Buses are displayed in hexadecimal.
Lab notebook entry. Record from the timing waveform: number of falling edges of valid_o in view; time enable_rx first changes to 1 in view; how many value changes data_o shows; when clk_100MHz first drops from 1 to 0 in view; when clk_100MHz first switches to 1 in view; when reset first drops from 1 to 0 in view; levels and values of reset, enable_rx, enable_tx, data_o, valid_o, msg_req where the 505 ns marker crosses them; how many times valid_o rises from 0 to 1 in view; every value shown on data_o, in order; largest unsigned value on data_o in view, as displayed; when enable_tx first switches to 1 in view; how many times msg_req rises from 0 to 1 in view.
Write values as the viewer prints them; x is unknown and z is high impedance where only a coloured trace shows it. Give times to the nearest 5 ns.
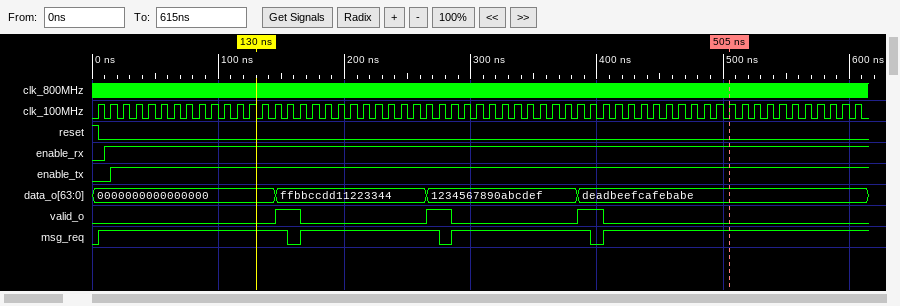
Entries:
3
10 ns
3
10 ns
5 ns
5 ns
reset=0, enable_rx=1, enable_tx=1, data_o=deadbeefcafebabe, valid_o=0, msg_req=1
3
0000000000000000, ffbbccdd11223344, 1234567890abcdef, deadbeefcafebabe
ffbbccdd11223344
15 ns
4
